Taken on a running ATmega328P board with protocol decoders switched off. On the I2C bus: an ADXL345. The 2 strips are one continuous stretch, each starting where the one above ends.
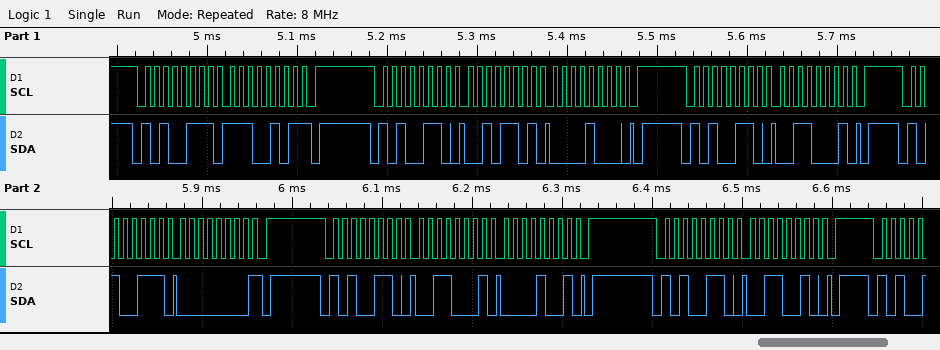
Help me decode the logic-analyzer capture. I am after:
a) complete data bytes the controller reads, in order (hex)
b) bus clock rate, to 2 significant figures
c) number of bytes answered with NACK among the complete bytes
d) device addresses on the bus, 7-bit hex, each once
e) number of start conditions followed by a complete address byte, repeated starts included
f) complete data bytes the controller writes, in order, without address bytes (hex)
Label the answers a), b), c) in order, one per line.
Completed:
a) E5 00
b) 100 kHz
c) 2
d) 0x53
e) 6
f) 2D 08 31 31 09 32
